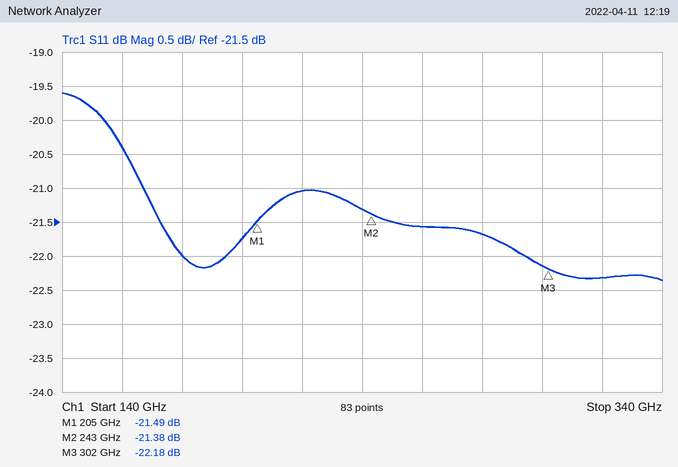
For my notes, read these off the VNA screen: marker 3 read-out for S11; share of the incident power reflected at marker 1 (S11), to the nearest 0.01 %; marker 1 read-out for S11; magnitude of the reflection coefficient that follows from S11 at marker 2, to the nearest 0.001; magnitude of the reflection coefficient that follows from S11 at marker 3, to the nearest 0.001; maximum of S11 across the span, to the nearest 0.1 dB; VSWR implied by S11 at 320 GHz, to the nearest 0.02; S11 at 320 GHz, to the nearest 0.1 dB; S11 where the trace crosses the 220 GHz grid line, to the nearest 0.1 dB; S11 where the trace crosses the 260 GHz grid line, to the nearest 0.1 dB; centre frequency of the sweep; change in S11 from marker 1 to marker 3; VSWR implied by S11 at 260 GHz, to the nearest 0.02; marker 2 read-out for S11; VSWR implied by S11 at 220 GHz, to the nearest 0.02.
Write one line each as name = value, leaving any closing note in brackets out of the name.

marker 3 read-out for S11 = -22.18 dB
share of the incident power reflected at marker 1 (S11), to the nearest 0.01 % = 0.71 %
marker 1 read-out for S11 = -21.49 dB
magnitude of the reflection coefficient that follows from S11 at marker 2, to the nearest 0.001 = 0.085
magnitude of the reflection coefficient that follows from S11 at marker 3, to the nearest 0.001 = 0.078
maximum of S11 across the span, to the nearest 0.1 dB = -19.6 dB
VSWR implied by S11 at 320 GHz, to the nearest 0.02 = 1.16
S11 at 320 GHz, to the nearest 0.1 dB = -22.3 dB
S11 where the trace crosses the 220 GHz grid line, to the nearest 0.1 dB = -21.0 dB
S11 where the trace crosses the 260 GHz grid line, to the nearest 0.1 dB = -21.6 dB
centre frequency of the sweep = 240 GHz
change in S11 from marker 1 to marker 3 = -0.69 dB
VSWR implied by S11 at 260 GHz, to the nearest 0.02 = 1.18
marker 2 read-out for S11 = -21.38 dB
VSWR implied by S11 at 220 GHz, to the nearest 0.02 = 1.20
